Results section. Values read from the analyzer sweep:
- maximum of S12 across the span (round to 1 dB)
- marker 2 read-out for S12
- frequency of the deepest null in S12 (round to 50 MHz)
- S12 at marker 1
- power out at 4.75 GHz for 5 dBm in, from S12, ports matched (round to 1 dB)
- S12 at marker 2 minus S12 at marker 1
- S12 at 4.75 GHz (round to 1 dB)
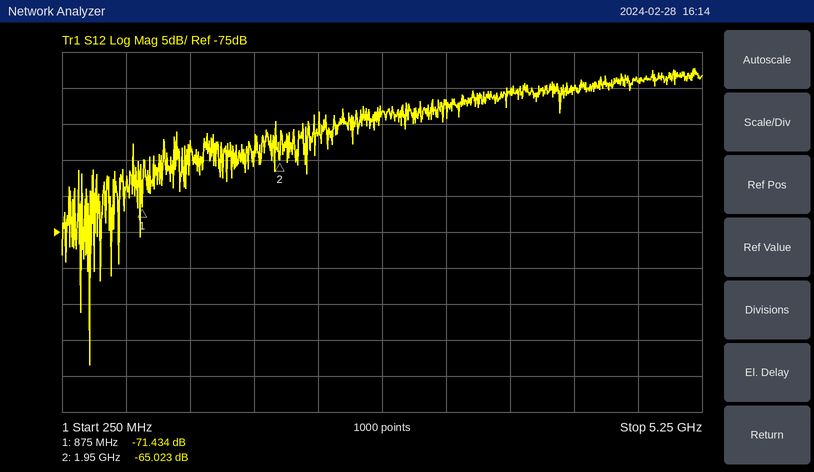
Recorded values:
-52 dB
-65.023 dB
450 MHz
-71.434 dB
-49 dBm
6.411 dB
-54 dB
